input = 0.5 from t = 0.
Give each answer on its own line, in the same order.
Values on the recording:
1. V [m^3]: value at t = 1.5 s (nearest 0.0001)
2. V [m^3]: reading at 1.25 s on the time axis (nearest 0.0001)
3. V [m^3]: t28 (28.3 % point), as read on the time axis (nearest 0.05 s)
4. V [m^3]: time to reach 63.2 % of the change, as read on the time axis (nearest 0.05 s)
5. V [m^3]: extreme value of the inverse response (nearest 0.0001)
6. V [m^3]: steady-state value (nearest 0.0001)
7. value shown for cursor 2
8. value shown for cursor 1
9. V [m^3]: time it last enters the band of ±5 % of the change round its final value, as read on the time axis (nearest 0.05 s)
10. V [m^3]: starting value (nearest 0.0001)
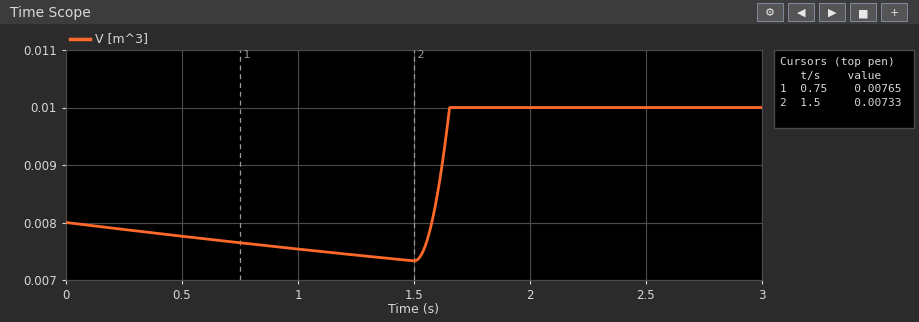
0.0073
0.0074
1.60 s
1.65 s
0.0073
0.0100
0.00733
0.00765
1.65 s
0.0080
